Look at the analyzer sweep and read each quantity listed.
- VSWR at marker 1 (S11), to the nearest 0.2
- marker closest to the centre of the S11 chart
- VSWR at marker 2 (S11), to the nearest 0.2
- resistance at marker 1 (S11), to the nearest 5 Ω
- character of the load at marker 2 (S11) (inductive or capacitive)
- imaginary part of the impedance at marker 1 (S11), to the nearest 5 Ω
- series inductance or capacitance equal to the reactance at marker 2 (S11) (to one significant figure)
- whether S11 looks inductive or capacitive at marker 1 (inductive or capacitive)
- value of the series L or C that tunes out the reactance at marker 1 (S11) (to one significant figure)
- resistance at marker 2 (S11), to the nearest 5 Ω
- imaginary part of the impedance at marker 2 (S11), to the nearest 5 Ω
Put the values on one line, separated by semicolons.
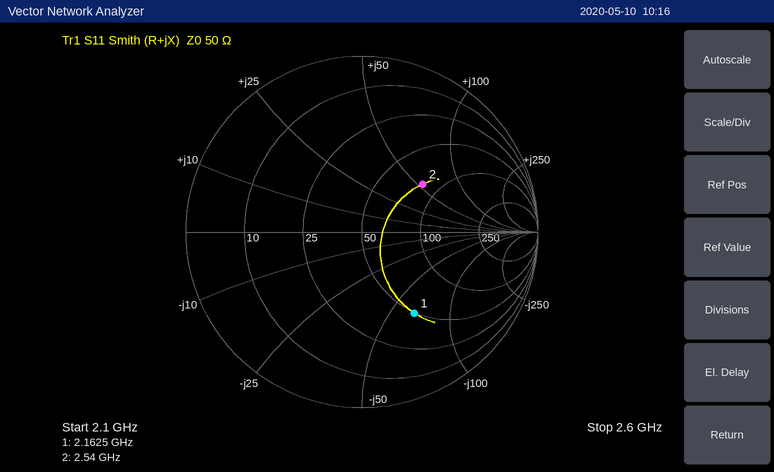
3.4; marker 2; 2.6; 50 Ω; inductive; -65 Ω; 3 nH; capacitive; 5 nH; 80 Ω; +55 Ω
